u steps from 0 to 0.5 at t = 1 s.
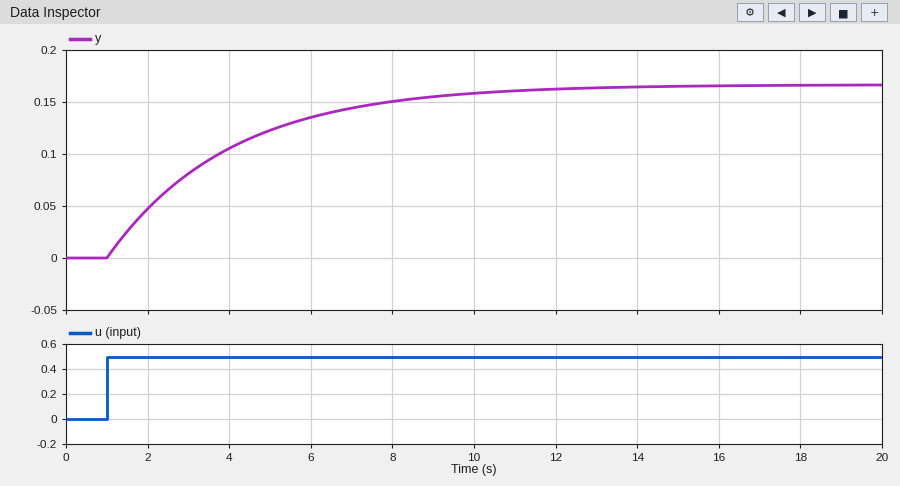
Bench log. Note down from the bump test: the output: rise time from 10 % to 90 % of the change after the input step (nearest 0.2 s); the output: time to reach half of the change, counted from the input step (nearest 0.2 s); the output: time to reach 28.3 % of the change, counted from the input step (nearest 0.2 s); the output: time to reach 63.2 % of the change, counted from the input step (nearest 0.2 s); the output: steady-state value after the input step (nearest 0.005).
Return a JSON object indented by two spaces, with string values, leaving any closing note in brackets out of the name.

{
  "the output: rise time from 10 % to 90 % of the change after the input step": "6.6 s",
  "the output: time to reach half of the change, counted from the input step": "2.0 s",
  "the output: time to reach 28.3 % of the change, counted from the input step": "1.0 s",
  "the output: time to reach 63.2 % of the change, counted from the input step": "3.0 s",
  "the output: steady-state value after the input step": "0.165"
}
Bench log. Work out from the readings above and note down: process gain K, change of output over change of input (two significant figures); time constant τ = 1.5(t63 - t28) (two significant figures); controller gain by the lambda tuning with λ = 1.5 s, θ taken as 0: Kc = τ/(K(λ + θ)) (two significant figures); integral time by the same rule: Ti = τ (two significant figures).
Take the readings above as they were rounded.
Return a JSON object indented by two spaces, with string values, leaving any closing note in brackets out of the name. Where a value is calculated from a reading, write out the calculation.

{
  "process gain K, change of output over change of input": "(0.165 - 0) / 0.5 = 0.33",
  "time constant τ = 1.5(t63 - t28)": "1.5 × (3 - 1) = 3.0 s",
  "controller gain by the lambda tuning with λ = 1.5 s, θ taken as 0: Kc = τ/(K(λ + θ))": "3 / (0.33 × (1.5 + 0)) = 6.1",
  "integral time by the same rule: Ti = τ": "3.0 s"
}
